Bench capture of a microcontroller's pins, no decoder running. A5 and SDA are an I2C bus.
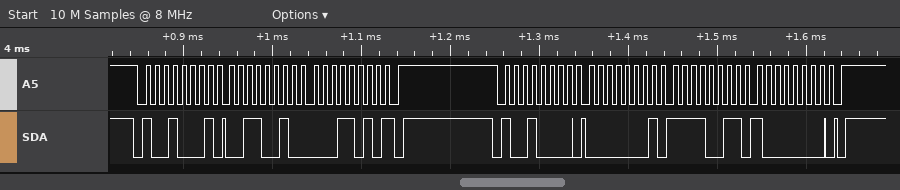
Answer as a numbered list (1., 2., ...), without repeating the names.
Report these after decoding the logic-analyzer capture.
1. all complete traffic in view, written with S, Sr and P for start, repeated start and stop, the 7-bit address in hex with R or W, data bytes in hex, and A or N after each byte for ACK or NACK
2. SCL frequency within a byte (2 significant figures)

1. S 48R A 32 A 1A N P S 48W A 01 A F3 A 80 A P
2. 100 kHz
